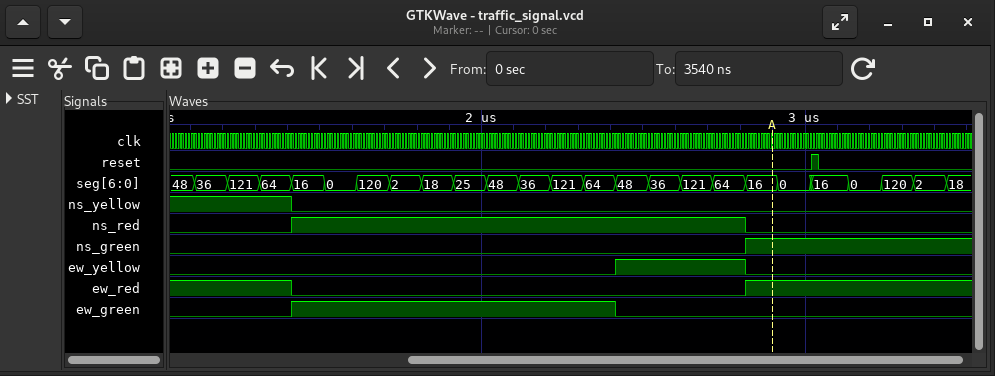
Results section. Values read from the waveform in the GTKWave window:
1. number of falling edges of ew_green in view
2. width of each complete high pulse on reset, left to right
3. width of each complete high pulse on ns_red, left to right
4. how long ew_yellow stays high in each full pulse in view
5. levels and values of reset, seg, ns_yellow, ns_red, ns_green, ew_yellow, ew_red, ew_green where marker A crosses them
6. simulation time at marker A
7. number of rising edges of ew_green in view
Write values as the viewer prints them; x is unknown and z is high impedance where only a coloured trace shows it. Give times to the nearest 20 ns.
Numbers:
1
20 ns
1400 ns
400 ns
reset=0, seg=16, ns_yellow=0, ns_red=0, ns_green=1, ew_yellow=0, ew_red=1, ew_green=0
2900 ns
1
